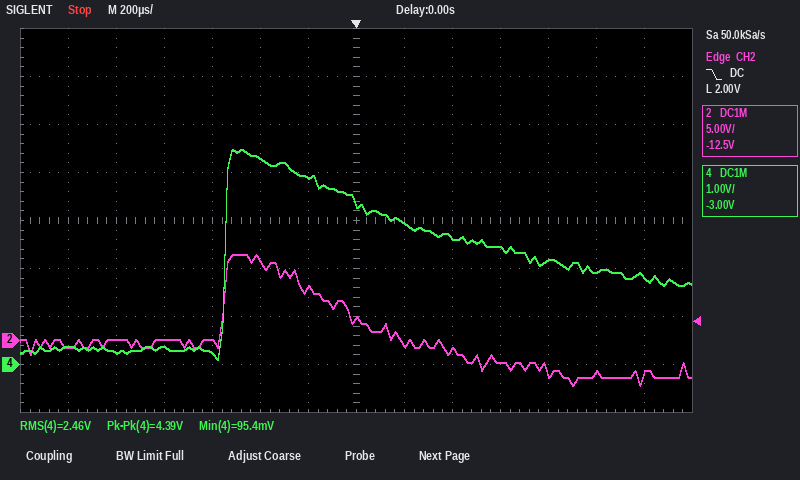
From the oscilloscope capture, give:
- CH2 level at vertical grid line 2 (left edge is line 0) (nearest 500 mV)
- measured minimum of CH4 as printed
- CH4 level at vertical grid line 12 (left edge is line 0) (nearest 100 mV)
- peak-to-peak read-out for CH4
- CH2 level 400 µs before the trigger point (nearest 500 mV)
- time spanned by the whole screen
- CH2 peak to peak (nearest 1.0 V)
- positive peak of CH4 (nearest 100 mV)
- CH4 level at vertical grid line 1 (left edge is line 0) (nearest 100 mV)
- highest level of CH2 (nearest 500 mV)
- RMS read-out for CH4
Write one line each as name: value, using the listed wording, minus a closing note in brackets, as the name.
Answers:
CH2 level at vertical grid line 2 (left edge is line 0): 0.0 V
measured minimum of CH4 as printed: 95.4 mV
CH4 level at vertical grid line 12 (left edge is line 0): 1.9 V
peak-to-peak read-out for CH4: 4.39 V
CH2 level 400 µs before the trigger point: 8.5 V
time spanned by the whole screen: 2.8 ms
CH2 peak to peak: 14.0 V
positive peak of CH4: 4.5 V
CH4 level at vertical grid line 1 (left edge is line 0): 400 mV
highest level of CH2: 9.0 V
RMS read-out for CH4: 2.46 V
